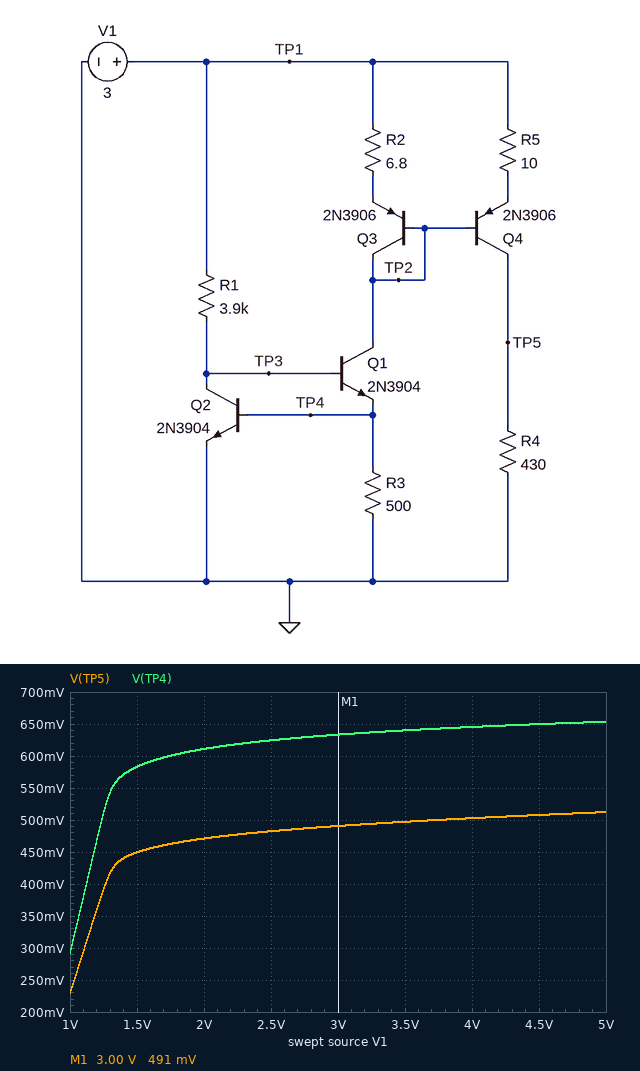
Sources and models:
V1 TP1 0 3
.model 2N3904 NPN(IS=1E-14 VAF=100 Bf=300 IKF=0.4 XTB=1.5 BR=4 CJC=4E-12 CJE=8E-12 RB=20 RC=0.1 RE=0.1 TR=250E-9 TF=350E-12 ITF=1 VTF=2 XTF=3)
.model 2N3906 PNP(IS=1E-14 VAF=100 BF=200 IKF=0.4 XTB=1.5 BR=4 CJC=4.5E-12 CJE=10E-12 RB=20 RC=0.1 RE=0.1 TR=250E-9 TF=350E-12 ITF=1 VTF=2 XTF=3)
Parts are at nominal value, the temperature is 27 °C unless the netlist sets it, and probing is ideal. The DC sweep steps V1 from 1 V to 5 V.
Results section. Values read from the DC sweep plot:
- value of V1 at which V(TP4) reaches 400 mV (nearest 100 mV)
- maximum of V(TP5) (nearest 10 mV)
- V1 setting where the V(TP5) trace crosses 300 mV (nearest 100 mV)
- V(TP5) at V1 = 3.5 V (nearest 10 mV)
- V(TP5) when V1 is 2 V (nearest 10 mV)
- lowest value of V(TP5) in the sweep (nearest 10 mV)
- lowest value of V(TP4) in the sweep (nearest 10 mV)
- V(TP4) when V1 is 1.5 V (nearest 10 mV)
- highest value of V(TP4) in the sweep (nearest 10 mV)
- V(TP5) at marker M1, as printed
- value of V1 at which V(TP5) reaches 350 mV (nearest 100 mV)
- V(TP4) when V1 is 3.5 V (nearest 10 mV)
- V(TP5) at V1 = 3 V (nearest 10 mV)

1.1 V
510 mV
1.1 V
500 mV
470 mV
230 mV
290 mV
580 mV
650 mV
491 mV
1.2 V
640 mV
490 mV
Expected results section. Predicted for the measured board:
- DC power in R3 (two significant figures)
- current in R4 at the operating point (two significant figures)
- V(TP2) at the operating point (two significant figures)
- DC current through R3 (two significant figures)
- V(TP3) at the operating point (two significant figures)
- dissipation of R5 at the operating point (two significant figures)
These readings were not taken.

800 µW
1.1 mA
2.3 V
1.3 mA
1.3 V
13 µW
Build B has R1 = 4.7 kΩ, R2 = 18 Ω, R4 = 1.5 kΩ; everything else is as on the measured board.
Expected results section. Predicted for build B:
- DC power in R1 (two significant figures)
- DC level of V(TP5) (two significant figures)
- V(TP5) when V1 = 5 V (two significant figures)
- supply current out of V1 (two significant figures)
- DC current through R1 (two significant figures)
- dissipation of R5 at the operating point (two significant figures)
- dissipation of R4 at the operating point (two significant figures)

620 µW
2.4 V
2.5 V
3.2 mA
360 µA
25 µW
3.8 mW
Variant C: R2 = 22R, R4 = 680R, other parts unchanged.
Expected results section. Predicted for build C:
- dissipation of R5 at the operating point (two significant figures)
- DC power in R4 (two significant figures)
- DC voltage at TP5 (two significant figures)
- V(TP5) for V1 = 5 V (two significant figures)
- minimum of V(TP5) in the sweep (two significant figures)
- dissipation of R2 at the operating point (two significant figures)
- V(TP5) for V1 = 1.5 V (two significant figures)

33 µW
2.2 mW
1.2 V
1.3 V
460 mV
35 µW
1.1 V
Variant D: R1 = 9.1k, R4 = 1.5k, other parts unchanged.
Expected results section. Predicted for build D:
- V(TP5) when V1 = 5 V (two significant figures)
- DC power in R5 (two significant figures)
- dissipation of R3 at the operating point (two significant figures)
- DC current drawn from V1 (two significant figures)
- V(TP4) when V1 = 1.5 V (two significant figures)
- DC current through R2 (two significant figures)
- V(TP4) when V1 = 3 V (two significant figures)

1.7 V
12 µW
750 µW
2.5 mA
560 mV
1.2 mA
610 mV
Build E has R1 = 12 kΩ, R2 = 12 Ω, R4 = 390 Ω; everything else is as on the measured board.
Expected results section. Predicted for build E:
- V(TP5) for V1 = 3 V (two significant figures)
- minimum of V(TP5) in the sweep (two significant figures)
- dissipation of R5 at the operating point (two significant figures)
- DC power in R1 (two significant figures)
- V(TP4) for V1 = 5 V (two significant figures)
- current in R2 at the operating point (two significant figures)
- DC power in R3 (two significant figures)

500 mV
210 mV
17 µW
250 µW
620 mV
1.2 mA
730 µW
